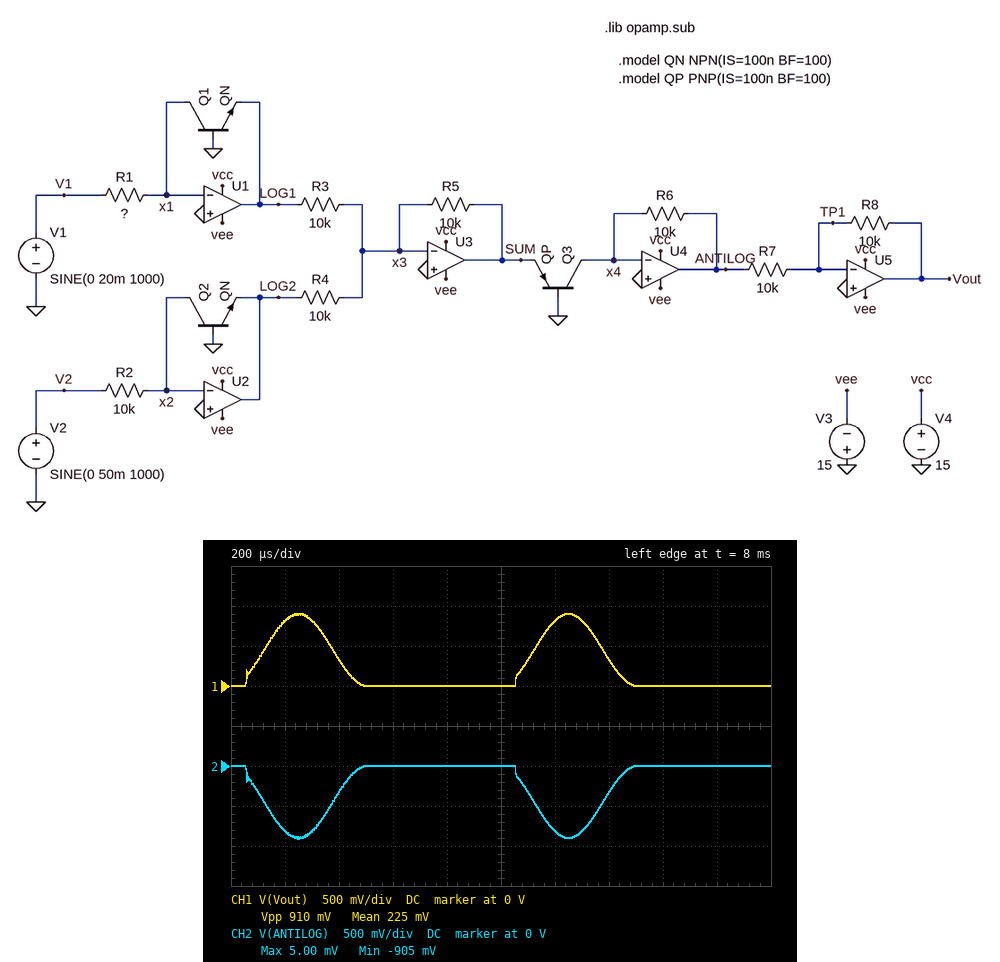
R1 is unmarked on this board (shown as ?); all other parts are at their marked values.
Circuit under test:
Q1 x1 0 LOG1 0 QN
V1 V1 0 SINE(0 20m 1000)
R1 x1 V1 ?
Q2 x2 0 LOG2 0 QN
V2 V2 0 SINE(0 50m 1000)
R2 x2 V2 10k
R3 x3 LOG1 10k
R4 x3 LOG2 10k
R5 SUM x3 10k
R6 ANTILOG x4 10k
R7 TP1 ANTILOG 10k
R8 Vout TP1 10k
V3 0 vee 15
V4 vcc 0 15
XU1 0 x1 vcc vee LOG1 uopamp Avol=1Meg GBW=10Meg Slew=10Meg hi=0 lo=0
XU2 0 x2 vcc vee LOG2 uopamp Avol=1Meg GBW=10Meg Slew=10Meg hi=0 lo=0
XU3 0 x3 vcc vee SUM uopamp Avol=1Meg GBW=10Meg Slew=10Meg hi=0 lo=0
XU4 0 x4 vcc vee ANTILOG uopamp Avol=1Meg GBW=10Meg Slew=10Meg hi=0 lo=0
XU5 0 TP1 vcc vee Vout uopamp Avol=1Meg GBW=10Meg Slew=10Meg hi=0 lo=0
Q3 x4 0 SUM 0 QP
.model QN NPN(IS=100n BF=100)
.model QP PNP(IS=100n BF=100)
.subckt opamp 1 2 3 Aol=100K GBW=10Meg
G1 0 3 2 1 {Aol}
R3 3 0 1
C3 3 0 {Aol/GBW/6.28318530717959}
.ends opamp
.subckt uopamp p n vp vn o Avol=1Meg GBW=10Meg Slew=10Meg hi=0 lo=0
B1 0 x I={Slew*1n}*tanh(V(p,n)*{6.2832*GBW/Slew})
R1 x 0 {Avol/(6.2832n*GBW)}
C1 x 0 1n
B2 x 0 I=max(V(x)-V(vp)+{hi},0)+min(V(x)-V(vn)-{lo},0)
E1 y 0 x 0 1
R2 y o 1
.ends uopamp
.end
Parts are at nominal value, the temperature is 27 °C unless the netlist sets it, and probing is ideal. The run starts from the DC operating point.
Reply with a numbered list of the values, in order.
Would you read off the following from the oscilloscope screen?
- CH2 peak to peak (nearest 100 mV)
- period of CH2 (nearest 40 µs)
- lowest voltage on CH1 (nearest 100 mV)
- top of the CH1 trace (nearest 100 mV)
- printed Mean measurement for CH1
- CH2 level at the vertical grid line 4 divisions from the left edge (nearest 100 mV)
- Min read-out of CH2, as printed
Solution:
1. 900 mV
2. 1.00 ms
3. 0 V
4. 900 mV
5. 225 mV
6. 0 V
7. -905 mV
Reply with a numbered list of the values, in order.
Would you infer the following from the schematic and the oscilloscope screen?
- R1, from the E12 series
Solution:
1. 12 kΩ
